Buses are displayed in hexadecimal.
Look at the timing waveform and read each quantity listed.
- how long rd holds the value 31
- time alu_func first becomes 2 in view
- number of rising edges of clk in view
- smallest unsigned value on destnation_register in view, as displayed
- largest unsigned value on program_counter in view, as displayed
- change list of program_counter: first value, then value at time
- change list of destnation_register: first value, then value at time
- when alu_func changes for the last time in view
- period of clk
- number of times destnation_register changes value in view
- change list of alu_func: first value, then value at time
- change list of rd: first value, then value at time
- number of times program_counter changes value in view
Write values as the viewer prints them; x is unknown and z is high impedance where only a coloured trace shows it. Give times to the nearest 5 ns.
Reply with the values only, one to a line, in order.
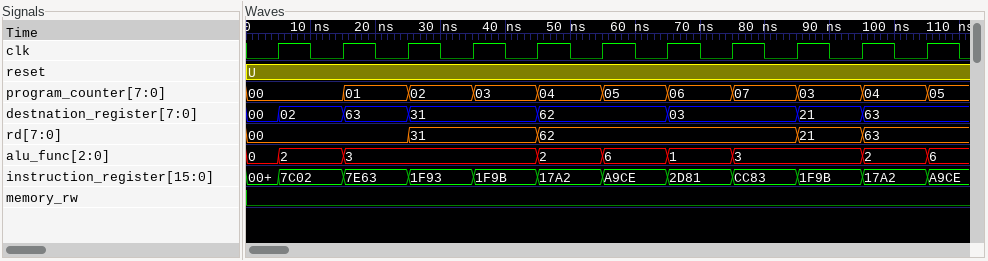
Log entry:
20 ns
5 ns
11
00
07
00, 01 at 15 ns, 02 at 25 ns, 03 at 35 ns, 04 at 45 ns, 05 at 55 ns, 06 at 65 ns, 07 at 75 ns, 03 at 85 ns, 04 at 95 ns, 05 at 105 ns
00, 02 at 5 ns, 63 at 15 ns, 31 at 25 ns, 62 at 45 ns, 03 at 65 ns, 21 at 85 ns, 63 at 95 ns
105 ns
10 ns
7
0, 2 at 5 ns, 3 at 15 ns, 2 at 45 ns, 6 at 55 ns, 1 at 65 ns, 3 at 75 ns, 2 at 95 ns, 6 at 105 ns
00, 31 at 25 ns, 62 at 45 ns, 21 at 85 ns, 63 at 95 ns
10
